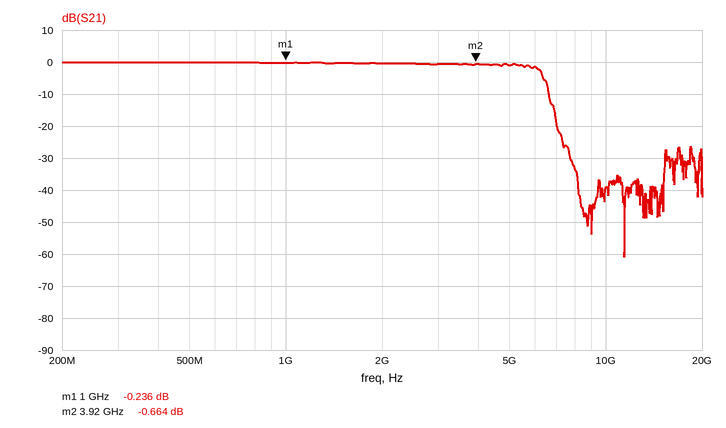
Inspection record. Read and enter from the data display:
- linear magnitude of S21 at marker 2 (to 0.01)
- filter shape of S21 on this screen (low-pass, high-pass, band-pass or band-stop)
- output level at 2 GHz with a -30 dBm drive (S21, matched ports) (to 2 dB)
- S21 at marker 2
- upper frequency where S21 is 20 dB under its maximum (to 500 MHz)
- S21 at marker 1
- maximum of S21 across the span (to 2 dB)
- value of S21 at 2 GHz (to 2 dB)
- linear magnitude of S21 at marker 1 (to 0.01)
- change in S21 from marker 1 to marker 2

0.93
low-pass
-30 dBm
-0.664 dB
7.0 GHz
-0.236 dB
0 dB
0 dB
0.97
-0.428 dB
